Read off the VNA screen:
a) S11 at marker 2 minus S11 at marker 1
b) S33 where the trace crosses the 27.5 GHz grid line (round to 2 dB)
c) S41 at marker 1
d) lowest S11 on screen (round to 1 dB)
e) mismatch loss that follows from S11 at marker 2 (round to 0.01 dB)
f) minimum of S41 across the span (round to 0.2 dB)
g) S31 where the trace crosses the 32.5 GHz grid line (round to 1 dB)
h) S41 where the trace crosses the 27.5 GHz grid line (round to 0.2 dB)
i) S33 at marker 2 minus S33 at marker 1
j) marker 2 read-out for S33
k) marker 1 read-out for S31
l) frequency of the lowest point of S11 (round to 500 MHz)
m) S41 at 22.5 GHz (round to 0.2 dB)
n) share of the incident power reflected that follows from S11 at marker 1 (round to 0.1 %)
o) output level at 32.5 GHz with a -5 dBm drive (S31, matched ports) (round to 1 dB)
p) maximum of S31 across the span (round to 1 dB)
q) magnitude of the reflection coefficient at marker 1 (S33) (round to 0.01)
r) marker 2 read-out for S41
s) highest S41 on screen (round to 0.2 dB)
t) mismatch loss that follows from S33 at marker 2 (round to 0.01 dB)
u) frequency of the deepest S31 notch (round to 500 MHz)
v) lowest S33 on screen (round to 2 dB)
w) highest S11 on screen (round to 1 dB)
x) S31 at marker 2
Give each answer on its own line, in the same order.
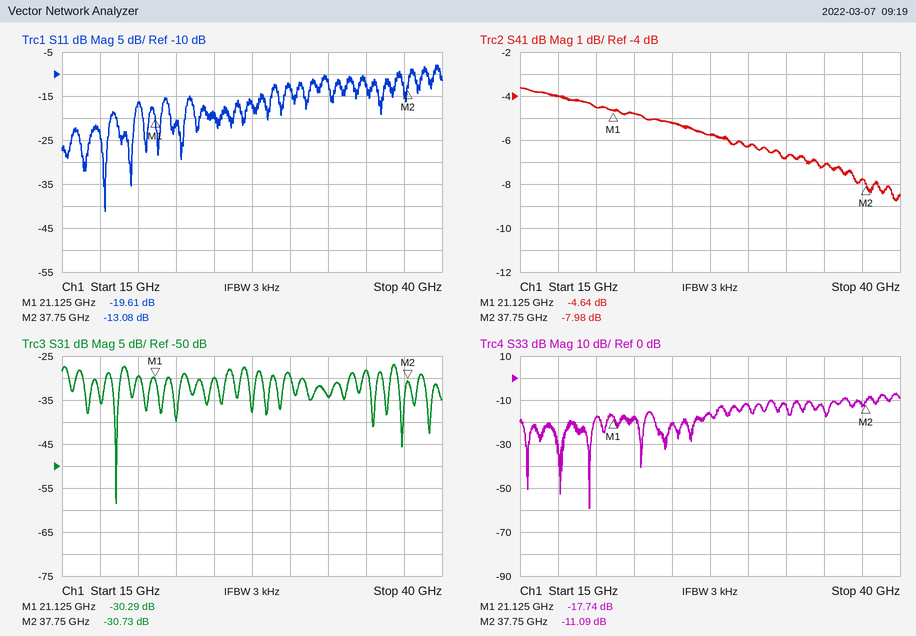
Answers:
6.53 dB
-16 dB
-4.64 dB
-41 dB
0.22 dB
-8.8 dB
-34 dB
-5.8 dB
6.65 dB
-11.09 dB
-30.29 dB
18.0 GHz
-4.8 dB
1.1 %
-39 dBm
-27 dB
0.13
-7.98 dB
-3.6 dB
0.35 dB
18.5 GHz
-60 dB
-8 dB
-30.73 dB
